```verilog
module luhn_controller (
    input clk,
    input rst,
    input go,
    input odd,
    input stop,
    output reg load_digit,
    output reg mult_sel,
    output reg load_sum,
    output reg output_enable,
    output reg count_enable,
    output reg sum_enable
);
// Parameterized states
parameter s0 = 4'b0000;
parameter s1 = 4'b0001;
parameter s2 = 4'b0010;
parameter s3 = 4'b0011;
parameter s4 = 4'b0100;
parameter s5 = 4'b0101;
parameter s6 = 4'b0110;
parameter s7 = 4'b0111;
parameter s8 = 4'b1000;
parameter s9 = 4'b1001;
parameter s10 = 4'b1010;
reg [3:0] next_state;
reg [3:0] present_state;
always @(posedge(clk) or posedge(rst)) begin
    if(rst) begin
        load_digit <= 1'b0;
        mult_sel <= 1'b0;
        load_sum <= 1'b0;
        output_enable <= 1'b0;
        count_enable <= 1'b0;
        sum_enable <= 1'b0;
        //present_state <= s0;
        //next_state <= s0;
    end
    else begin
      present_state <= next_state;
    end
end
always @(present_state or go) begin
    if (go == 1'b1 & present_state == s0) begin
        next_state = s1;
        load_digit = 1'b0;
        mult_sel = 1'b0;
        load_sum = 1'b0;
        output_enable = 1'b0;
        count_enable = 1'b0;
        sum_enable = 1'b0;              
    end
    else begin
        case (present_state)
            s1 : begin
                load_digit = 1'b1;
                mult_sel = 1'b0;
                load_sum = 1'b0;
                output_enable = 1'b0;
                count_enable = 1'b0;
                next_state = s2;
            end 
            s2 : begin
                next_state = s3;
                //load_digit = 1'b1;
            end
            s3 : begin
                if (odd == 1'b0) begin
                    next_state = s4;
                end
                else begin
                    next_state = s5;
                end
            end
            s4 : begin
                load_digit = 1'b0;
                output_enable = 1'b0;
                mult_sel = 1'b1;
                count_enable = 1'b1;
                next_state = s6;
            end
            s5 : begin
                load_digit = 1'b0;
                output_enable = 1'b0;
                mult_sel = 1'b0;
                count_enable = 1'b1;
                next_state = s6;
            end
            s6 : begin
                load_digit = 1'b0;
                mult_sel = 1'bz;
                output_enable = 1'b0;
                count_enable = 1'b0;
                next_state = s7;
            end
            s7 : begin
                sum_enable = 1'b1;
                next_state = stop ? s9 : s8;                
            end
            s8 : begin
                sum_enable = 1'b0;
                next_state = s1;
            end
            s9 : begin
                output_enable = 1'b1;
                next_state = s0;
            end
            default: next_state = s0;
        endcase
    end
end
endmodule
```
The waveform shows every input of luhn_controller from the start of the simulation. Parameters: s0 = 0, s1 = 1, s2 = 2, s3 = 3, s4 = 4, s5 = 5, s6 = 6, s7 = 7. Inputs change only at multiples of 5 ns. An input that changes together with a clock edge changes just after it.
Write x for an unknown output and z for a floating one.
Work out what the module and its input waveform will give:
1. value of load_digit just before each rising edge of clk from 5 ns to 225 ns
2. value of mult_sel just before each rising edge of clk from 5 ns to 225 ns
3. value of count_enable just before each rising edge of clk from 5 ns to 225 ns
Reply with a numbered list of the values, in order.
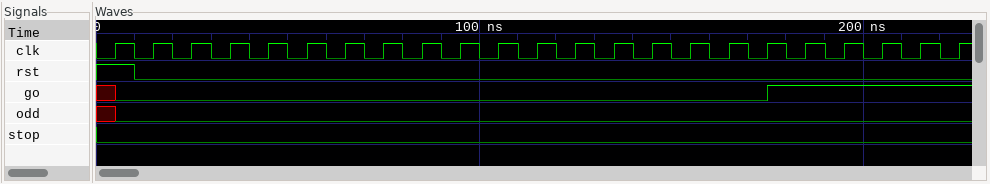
1. 0 0 0 0 0 0 0 0 0 0 0 0 0 0 0 0 0 0 0 1 1 1 0
2. 0 0 0 0 0 0 0 0 0 0 0 0 0 0 0 0 0 0 0 0 0 0 1
3. 0 0 0 0 0 0 0 0 0 0 0 0 0 0 0 0 0 0 0 0 0 0 1
